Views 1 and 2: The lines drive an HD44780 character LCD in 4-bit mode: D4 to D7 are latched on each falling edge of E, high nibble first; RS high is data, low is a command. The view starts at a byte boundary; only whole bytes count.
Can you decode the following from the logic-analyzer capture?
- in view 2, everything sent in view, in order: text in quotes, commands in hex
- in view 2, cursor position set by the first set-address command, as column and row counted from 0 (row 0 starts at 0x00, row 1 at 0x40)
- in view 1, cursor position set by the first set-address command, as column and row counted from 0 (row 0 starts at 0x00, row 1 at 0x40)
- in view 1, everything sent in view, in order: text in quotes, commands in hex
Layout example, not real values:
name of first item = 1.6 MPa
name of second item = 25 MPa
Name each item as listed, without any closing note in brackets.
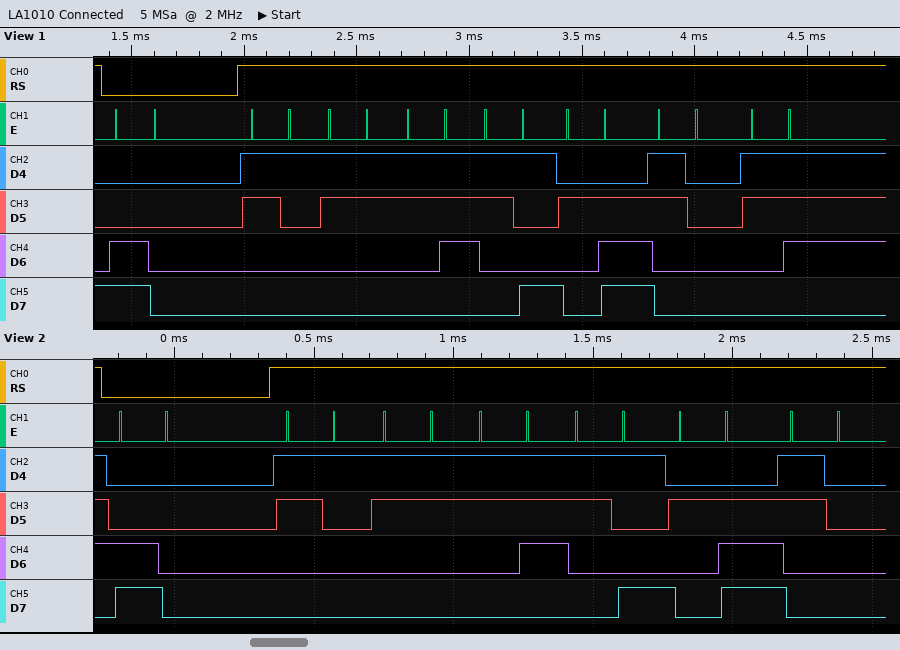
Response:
in view 2, everything sent in view, in order: text in quotes, commands in hex = 0xC0 "1379.0"
in view 2, cursor position set by the first set-address command, as column and row counted from 0 = column 0, row 1
in view 1, cursor position set by the first set-address command, as column and row counted from 0 = column 0, row 1
in view 1, everything sent in view, in order: text in quotes, commands in hex = 0xC0 "1379.07"
